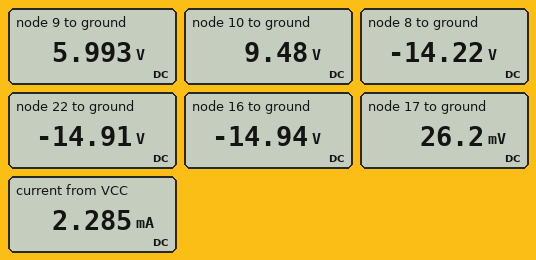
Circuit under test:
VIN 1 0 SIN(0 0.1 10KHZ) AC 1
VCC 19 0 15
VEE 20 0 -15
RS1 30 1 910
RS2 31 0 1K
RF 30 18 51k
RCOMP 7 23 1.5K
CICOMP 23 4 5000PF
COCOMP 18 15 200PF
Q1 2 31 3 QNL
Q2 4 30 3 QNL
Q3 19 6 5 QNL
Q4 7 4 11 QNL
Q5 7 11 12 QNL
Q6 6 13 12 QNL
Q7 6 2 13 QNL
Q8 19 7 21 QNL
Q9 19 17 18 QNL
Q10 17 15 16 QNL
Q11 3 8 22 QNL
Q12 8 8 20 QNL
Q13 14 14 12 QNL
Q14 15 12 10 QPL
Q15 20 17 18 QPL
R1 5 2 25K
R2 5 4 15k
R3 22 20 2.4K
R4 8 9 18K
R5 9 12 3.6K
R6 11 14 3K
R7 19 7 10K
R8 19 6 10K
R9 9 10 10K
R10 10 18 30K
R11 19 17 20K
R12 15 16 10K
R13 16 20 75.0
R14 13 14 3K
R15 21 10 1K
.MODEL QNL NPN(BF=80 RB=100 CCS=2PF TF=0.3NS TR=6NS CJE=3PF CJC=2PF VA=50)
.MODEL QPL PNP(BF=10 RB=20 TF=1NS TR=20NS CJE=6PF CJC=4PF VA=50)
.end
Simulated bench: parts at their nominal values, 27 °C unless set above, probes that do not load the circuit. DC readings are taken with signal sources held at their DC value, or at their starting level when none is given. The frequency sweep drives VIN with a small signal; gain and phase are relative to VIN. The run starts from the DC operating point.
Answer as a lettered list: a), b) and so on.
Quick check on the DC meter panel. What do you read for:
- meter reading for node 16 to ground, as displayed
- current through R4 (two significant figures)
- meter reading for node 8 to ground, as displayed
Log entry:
a) -14.94 V
b) 1.1 mA
c) -14.22 V
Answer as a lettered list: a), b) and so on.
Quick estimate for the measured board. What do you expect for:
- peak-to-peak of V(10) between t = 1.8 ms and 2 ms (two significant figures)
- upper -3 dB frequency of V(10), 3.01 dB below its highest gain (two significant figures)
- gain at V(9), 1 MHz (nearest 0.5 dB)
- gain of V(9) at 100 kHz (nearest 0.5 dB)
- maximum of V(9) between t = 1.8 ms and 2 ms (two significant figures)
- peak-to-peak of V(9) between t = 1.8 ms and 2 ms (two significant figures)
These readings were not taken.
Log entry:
a) 130 mV
b) 4.6 MHz
c) -0.5 dB
d) -13.0 dB
e) 6.1 V
f) 120 mV
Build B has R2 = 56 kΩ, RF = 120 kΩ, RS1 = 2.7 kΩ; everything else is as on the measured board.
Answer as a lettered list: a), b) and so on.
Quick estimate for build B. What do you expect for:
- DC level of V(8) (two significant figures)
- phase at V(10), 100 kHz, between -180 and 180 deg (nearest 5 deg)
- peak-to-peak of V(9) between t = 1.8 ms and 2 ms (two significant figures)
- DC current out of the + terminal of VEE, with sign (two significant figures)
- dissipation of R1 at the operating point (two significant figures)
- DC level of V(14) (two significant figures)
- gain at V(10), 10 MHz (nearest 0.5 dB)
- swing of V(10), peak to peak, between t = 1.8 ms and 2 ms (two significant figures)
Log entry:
a) -14 V
b) 5 deg
c) 160 mV
d) -2.4 mA
e) 18 µW
f) 9.3 V
g) -7.0 dB
h) 190 mV
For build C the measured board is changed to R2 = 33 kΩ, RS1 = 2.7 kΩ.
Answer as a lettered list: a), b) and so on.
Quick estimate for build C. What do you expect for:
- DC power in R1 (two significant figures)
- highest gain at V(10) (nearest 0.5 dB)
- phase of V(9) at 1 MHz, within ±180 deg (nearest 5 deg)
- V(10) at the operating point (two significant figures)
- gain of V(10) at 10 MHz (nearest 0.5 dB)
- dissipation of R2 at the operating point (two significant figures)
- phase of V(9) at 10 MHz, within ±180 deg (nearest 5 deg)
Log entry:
a) 12 µW
b) 5.0 dB
c) -5 deg
d) 9.4 V
e) -6.5 dB
f) 9.2 µW
g) -150 deg
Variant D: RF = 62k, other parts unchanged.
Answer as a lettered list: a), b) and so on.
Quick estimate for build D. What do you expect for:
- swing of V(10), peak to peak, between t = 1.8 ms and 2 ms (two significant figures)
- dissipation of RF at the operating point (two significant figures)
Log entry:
a) 140 mV
b) 13 µW
